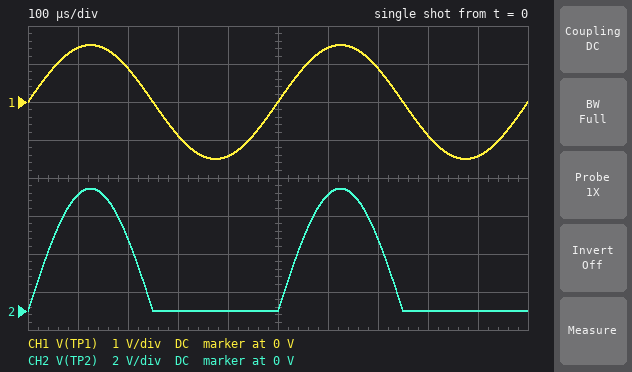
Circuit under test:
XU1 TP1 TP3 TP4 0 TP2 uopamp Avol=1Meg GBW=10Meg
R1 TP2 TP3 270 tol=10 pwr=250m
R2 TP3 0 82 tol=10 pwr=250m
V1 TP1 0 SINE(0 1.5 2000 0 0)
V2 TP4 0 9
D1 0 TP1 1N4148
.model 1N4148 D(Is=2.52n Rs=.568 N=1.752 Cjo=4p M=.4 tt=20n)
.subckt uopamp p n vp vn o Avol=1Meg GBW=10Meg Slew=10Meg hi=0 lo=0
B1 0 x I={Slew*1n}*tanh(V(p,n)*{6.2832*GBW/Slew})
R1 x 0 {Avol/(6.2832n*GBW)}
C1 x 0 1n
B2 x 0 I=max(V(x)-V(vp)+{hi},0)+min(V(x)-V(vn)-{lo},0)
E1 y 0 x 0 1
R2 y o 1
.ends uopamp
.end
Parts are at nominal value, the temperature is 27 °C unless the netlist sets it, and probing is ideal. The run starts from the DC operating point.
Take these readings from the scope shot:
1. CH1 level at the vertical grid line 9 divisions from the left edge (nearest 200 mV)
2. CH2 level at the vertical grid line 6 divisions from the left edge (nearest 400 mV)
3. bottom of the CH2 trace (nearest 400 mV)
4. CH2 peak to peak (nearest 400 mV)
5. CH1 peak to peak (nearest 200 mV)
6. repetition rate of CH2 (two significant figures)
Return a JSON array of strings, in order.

["-1.4 V", "6.0 V", "0 V", "6.4 V", "3.0 V", "2.0 kHz"]
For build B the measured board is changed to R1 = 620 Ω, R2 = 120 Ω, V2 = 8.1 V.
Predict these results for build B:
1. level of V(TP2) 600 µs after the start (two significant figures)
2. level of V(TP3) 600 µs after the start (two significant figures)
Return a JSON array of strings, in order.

["8.1 V", "1.3 V"]
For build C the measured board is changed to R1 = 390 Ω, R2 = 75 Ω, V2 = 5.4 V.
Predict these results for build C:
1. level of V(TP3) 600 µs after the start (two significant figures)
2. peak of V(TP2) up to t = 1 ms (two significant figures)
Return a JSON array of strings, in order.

["870 mV", "5.4 V"]
